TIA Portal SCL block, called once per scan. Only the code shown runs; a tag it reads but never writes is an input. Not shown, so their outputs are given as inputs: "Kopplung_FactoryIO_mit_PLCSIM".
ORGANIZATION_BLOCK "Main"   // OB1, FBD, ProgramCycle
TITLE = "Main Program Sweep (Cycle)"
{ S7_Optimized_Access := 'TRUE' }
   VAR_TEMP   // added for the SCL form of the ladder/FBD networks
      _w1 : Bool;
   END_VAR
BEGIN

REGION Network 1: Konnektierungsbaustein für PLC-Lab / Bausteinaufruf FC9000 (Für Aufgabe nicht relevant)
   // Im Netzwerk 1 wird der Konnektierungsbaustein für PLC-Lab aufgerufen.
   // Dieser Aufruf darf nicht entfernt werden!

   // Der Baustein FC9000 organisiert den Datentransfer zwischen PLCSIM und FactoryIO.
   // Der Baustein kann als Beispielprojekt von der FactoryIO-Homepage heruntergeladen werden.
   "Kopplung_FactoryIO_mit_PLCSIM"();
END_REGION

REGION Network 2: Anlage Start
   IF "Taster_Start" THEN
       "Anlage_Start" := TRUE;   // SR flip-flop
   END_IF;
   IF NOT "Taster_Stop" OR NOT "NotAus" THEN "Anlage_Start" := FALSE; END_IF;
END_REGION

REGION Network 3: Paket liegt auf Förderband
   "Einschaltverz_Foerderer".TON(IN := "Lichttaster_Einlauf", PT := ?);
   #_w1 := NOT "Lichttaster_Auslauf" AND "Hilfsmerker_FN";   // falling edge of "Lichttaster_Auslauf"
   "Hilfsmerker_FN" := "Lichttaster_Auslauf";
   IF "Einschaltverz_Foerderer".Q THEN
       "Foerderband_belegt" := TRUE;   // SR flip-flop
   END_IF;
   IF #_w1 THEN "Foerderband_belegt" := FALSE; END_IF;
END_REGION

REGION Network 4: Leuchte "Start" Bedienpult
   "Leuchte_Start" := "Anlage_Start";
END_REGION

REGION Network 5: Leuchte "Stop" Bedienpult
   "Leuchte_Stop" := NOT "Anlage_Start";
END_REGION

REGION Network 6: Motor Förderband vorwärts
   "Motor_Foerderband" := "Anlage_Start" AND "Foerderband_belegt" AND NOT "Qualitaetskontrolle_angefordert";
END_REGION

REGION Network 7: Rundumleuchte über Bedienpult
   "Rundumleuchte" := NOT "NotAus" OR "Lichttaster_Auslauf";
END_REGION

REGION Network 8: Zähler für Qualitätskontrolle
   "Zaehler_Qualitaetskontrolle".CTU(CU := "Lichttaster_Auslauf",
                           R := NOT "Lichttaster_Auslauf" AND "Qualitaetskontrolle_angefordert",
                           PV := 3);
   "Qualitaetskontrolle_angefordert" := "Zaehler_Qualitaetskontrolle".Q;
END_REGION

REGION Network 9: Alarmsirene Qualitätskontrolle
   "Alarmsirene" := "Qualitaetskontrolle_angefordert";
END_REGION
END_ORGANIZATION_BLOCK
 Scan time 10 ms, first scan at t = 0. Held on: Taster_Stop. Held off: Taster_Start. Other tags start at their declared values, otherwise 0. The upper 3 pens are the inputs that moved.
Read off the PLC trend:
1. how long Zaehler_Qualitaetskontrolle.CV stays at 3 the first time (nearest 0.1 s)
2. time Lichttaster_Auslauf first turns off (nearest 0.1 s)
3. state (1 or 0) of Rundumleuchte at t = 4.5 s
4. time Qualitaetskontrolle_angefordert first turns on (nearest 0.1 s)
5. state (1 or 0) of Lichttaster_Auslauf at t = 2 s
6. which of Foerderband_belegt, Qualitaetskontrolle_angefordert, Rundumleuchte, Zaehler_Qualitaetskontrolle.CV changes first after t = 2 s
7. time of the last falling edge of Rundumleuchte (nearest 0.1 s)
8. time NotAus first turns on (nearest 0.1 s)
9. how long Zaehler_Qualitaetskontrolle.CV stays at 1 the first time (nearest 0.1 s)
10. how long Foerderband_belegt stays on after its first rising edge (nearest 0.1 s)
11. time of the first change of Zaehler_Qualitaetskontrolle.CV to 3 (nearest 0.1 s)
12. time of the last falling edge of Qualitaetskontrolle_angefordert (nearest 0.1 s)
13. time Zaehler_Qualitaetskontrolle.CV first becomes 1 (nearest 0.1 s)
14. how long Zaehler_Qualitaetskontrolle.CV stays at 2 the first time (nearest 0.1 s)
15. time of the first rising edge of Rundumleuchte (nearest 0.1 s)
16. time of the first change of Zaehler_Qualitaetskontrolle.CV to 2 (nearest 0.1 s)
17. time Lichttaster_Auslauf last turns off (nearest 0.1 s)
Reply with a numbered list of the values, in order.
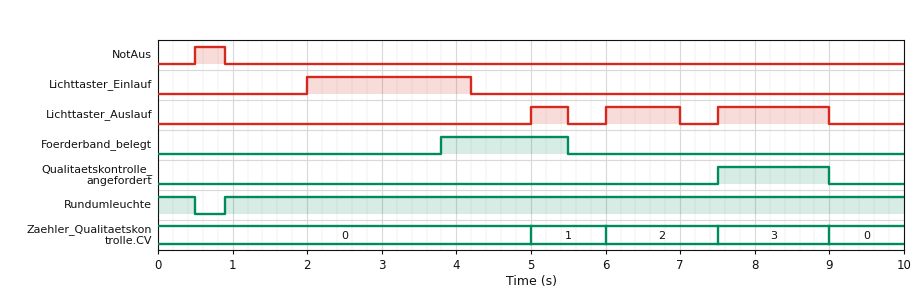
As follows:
1. 1.5 s
2. 5.5 s
3. 1
4. 7.5 s
5. 0
6. Foerderband_belegt
7. 0.5 s
8. 0.5 s
9. 1.0 s
10. 1.7 s
11. 7.5 s
12. 9.0 s
13. 5.0 s
14. 1.5 s
15. 0.9 s
16. 6.0 s
17. 9.0 s
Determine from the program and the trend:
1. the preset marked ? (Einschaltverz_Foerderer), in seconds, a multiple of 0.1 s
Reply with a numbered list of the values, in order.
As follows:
1. 1.8 s
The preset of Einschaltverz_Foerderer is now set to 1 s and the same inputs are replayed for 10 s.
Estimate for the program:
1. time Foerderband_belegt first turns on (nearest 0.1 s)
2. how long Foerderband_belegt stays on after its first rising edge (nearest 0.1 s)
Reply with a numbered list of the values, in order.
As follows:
1. 3.0 s
2. 2.5 s
